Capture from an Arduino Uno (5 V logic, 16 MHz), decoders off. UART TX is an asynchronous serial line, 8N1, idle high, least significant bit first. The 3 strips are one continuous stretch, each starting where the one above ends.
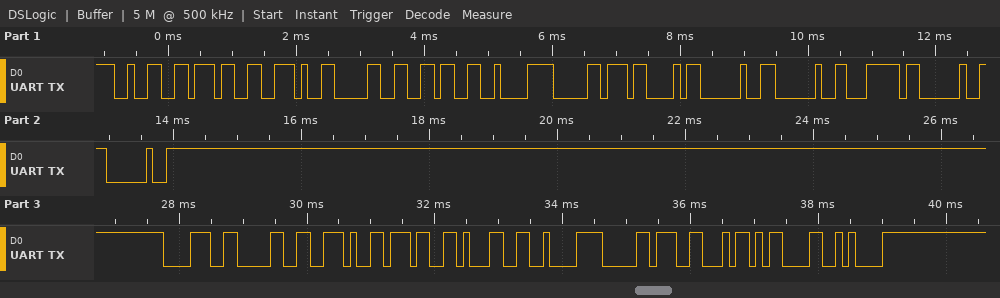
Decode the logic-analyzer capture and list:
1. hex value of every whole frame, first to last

32 37 2E 30 36 C2 B0 43 20 20 7C 20 20 38 30 2E 37 31 C2 B0 46 0D 0A
